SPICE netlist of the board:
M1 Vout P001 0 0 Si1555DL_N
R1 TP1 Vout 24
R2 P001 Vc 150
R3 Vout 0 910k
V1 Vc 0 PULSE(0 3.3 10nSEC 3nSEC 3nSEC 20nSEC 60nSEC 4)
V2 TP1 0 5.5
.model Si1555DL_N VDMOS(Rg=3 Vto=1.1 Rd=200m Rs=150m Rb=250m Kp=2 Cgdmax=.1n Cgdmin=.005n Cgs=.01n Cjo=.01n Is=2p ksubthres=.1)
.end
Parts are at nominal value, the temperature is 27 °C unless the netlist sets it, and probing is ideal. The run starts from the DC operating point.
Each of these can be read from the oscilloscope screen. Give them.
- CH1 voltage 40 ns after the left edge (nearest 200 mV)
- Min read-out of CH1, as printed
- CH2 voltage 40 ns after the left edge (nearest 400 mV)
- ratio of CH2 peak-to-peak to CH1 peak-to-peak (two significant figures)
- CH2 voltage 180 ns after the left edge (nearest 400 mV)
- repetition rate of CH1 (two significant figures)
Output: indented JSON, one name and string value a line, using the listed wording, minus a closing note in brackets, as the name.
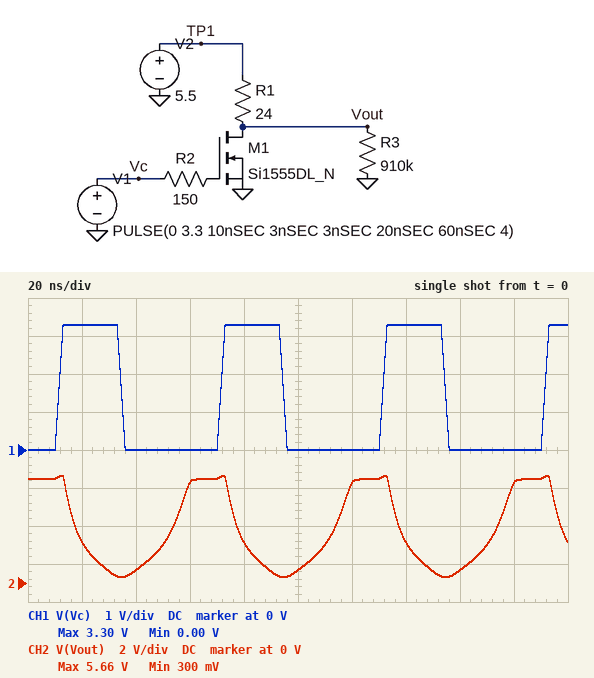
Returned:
{
  "CH1 voltage 40 ns after the left edge": "0 V",
  "Min read-out of CH1, as printed": "0.00 V",
  "CH2 voltage 40 ns after the left edge": "800 mV",
  "ratio of CH2 peak-to-peak to CH1 peak-to-peak": "1.6",
  "CH2 voltage 180 ns after the left edge": "5.2 V",
  "repetition rate of CH1": "17 MHz"
}
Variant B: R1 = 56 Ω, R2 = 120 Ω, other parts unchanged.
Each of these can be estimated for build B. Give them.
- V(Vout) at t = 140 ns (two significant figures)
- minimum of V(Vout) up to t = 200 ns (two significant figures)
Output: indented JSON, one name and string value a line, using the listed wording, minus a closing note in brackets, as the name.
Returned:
{
  "V(Vout) at t = 140 ns": "1.5 V",
  "minimum of V(Vout) up to t = 200 ns": "81 mV"
}
